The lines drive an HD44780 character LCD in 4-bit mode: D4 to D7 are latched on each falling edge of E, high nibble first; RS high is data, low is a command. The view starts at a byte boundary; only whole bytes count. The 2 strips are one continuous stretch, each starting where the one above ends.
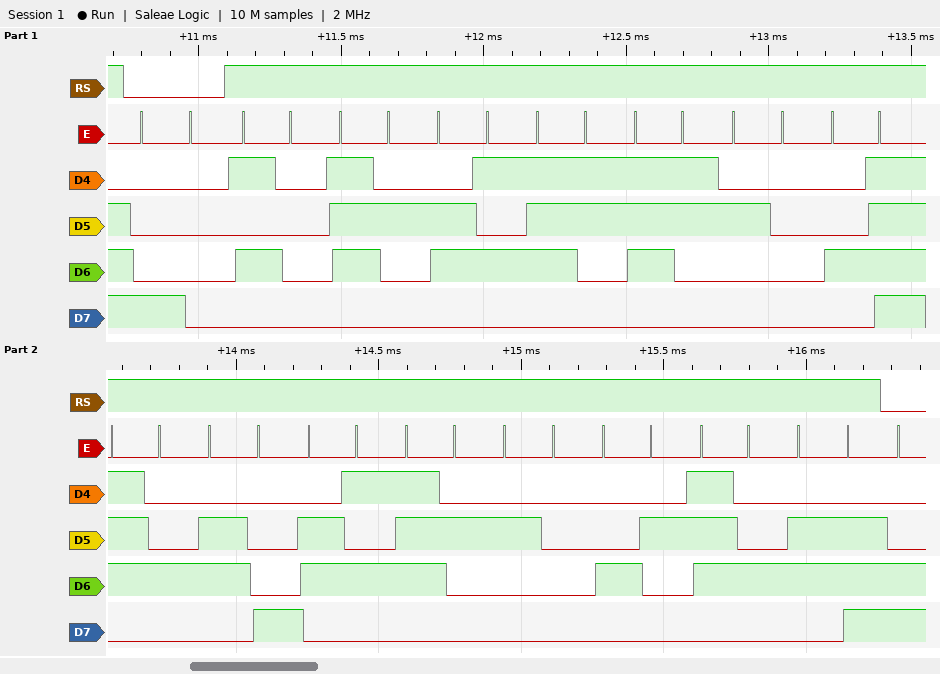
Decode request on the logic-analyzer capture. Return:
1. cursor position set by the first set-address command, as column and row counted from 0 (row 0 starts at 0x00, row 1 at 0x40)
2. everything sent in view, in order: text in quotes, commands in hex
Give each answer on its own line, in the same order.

column 0, row 0
0x80 "Press Other Btn"
